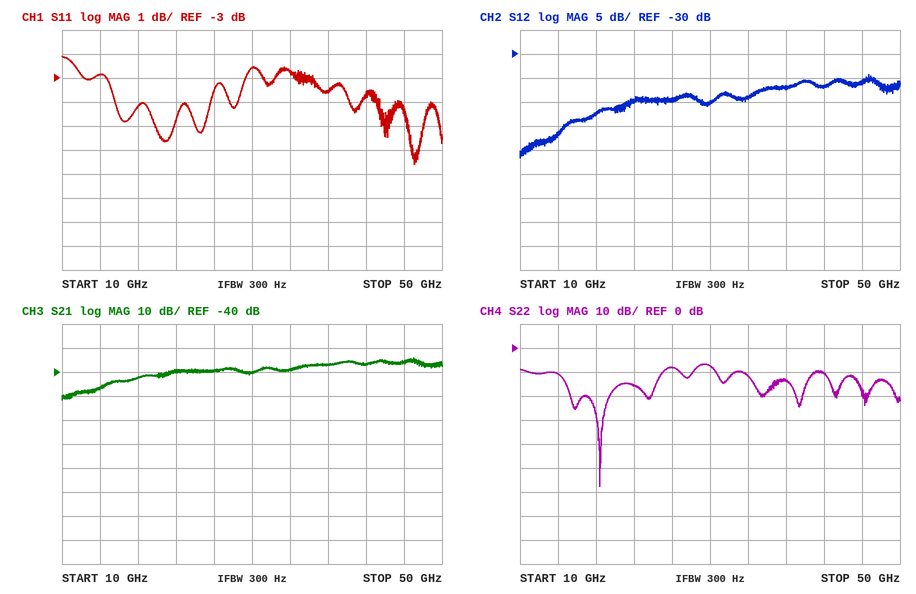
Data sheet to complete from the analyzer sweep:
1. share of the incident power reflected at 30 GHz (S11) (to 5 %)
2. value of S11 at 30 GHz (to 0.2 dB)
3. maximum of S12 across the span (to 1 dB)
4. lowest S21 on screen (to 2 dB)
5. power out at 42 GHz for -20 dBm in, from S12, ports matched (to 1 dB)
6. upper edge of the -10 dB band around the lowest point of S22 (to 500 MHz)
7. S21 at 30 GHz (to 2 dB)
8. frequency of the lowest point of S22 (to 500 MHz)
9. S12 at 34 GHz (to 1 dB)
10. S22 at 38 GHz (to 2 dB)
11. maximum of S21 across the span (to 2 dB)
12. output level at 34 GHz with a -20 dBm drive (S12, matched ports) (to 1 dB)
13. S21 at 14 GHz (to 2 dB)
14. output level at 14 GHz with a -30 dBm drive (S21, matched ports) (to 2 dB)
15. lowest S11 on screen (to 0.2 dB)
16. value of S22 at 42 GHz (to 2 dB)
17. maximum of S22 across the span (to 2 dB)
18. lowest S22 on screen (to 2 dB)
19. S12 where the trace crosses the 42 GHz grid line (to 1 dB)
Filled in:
55 %
-2.6 dB
-34 dB
-52 dB
-57 dBm
25.0 GHz
-40 dB
18.5 GHz
-39 dB
-14 dB
-34 dB
-59 dBm
-46 dB
-76 dBm
-6.6 dB
-10 dB
-6 dB
-58 dB
-37 dB
